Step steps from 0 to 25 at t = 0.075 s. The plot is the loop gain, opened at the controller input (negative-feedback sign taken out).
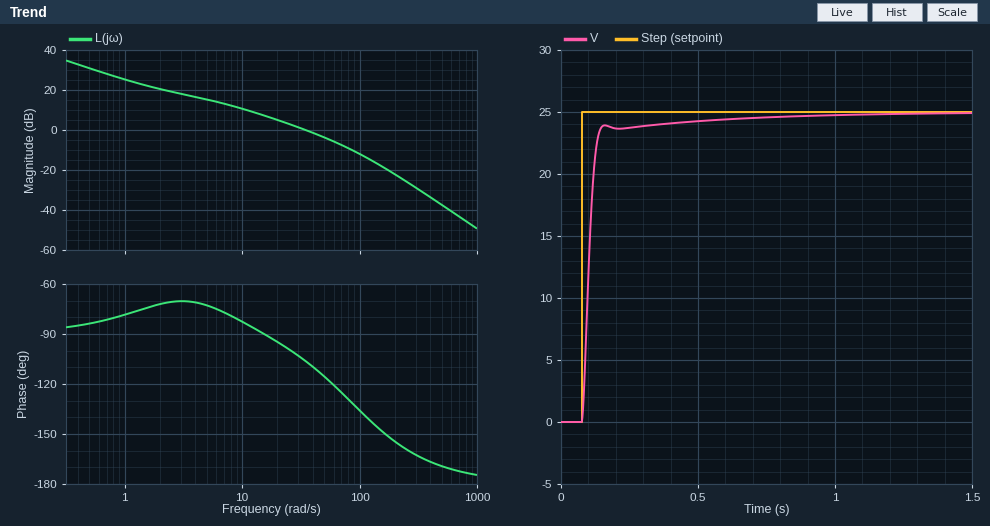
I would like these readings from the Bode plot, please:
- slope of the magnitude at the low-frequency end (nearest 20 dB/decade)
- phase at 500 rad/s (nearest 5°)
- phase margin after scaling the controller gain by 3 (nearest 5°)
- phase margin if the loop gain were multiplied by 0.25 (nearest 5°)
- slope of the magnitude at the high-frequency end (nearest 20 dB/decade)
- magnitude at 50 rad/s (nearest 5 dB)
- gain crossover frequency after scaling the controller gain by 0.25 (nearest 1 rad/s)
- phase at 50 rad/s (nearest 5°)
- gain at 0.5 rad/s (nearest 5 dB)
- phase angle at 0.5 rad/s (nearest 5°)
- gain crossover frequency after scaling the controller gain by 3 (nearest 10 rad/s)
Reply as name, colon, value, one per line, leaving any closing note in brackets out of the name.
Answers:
slope of the magnitude at the low-frequency end: -20 dB/decade
phase at 500 rad/s: -170°
phase margin after scaling the controller gain by 3: 50°
phase margin if the loop gain were multiplied by 0.25: 100°
slope of the magnitude at the high-frequency end: -40 dB/decade
magnitude at 50 rad/s: -5 dB
gain crossover frequency after scaling the controller gain by 0.25: 8 rad/s
phase at 50 rad/s: -115°
gain at 0.5 rad/s: 30 dB
phase angle at 0.5 rad/s: -85°
gain crossover frequency after scaling the controller gain by 3: 80 rad/s
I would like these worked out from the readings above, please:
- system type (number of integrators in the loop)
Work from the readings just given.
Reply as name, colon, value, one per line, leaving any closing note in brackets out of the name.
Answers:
system type: 1
